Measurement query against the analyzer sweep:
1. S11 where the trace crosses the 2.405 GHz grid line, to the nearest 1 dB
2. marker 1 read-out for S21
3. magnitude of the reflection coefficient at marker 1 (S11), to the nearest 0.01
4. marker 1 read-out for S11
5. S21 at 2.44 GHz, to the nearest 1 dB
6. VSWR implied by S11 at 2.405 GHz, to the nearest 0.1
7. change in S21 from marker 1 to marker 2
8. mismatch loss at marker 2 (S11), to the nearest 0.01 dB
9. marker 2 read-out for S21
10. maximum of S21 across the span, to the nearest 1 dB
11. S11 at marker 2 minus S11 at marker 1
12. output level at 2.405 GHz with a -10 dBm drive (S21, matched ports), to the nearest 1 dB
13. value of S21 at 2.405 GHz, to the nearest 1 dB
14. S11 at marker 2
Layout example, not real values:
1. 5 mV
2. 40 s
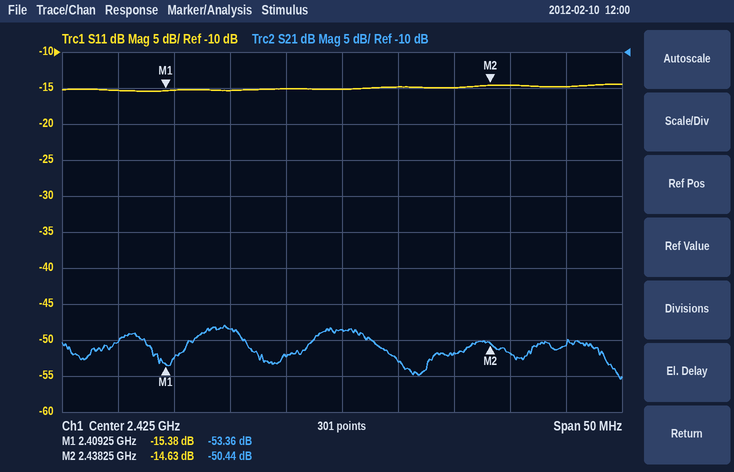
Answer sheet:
1. -15 dB
2. -53.36 dB
3. 0.17
4. -15.38 dB
5. -52 dB
6. 1.4
7. 2.92 dB
8. 0.15 dB
9. -50.44 dB
10. -48 dB
11. 0.75 dB
12. -60 dBm
13. -50 dB
14. -14.63 dB
